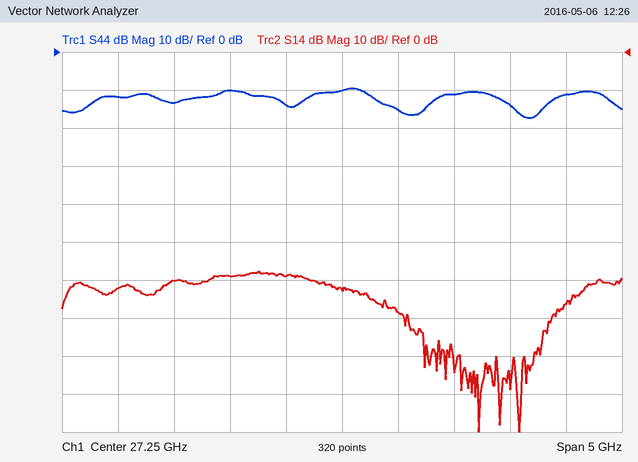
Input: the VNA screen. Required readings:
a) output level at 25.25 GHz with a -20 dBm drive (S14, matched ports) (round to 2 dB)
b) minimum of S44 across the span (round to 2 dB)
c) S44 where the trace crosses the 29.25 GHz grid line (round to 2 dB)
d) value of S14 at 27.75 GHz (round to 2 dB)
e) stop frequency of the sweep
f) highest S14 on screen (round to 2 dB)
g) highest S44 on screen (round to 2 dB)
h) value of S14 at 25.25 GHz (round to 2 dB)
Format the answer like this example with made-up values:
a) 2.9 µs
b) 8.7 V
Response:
a) -82 dBm
b) -18 dB
c) -12 dB
d) -68 dB
e) 29.75 GHz
f) -58 dB
g) -10 dB
h) -62 dB
